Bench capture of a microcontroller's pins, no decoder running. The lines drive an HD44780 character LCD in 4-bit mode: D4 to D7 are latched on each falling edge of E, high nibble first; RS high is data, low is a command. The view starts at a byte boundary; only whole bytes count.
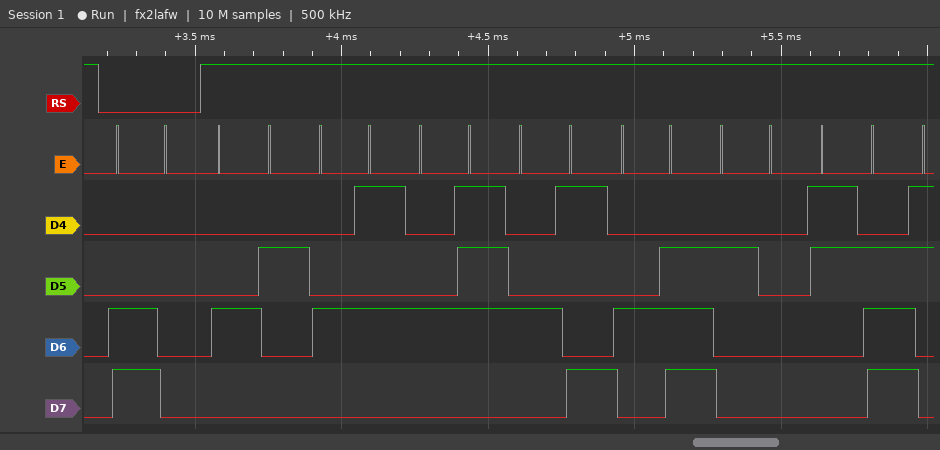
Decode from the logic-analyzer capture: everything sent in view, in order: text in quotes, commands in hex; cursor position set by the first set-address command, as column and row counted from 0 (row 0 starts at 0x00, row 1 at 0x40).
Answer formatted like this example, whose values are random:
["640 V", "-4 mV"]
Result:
["0xC0 \"BEGIN >\"", "column 0, row 1"]
